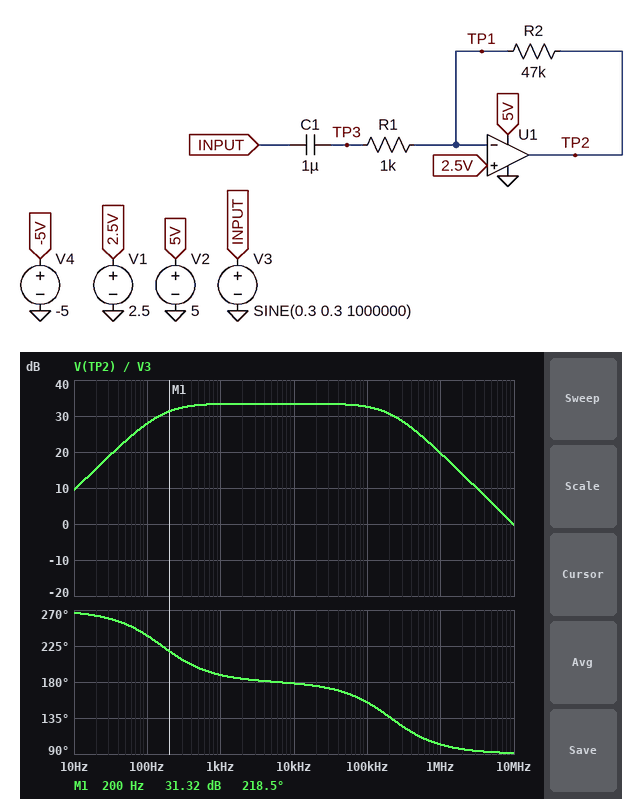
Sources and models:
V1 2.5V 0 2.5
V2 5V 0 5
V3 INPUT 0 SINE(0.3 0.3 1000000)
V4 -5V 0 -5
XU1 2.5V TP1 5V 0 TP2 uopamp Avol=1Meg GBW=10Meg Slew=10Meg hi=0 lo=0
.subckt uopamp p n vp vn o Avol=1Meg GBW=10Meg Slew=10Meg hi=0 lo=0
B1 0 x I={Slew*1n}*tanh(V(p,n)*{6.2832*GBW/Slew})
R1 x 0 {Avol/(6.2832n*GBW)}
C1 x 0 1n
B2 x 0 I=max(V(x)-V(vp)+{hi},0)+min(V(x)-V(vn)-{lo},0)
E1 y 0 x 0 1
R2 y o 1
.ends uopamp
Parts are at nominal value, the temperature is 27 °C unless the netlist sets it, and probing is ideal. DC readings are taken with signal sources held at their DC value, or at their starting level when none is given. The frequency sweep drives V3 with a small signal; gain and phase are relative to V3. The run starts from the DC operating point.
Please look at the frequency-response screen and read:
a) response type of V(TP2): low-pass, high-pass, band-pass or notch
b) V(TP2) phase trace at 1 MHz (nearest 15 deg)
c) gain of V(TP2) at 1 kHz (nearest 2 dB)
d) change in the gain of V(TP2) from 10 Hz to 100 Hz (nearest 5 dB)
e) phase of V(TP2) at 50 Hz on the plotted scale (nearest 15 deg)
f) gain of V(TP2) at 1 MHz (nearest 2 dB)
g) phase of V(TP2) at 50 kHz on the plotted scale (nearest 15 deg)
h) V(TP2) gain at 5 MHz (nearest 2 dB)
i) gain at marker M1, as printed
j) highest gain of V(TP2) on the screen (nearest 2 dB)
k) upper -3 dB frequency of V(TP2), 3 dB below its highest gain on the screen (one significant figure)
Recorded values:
band-pass
105 deg
34 dB
20 dB
255 deg
20 dB
165 deg
6 dB
31.32 dB
34 dB
200 kHz
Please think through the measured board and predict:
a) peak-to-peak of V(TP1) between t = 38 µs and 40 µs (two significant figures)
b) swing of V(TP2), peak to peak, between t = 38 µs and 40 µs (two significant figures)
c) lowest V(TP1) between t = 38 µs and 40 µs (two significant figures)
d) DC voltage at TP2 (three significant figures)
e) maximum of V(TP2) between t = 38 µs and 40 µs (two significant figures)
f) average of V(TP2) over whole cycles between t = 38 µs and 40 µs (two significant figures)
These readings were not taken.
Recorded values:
580 mV
3.7 V
2.2 V
2.50 V
4.3 V
2.5 V
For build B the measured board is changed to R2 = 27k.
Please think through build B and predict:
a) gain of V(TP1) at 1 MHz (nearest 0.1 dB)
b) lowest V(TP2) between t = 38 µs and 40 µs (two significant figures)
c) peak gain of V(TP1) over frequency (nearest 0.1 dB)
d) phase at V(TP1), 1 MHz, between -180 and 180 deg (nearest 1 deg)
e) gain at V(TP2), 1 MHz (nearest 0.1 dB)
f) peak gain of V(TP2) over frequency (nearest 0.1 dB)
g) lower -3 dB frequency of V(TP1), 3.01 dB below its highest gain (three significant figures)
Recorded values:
-0.8 dB
690 mV
-0.3 dB
20 deg
19.2 dB
28.6 dB
357 kHz
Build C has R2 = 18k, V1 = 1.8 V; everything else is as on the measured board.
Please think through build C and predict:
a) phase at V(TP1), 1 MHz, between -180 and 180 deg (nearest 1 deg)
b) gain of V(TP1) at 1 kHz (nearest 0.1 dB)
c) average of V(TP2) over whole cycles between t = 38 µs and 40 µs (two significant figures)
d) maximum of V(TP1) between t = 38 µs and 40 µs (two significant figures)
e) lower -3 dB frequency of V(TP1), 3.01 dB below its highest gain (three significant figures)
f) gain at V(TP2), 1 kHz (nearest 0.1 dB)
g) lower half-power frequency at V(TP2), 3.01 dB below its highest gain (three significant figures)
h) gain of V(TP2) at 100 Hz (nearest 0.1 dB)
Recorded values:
28 deg
-55.0 dB
1.8 V
2.1 V
526 kHz
25.0 dB
159 Hz
19.6 dB
